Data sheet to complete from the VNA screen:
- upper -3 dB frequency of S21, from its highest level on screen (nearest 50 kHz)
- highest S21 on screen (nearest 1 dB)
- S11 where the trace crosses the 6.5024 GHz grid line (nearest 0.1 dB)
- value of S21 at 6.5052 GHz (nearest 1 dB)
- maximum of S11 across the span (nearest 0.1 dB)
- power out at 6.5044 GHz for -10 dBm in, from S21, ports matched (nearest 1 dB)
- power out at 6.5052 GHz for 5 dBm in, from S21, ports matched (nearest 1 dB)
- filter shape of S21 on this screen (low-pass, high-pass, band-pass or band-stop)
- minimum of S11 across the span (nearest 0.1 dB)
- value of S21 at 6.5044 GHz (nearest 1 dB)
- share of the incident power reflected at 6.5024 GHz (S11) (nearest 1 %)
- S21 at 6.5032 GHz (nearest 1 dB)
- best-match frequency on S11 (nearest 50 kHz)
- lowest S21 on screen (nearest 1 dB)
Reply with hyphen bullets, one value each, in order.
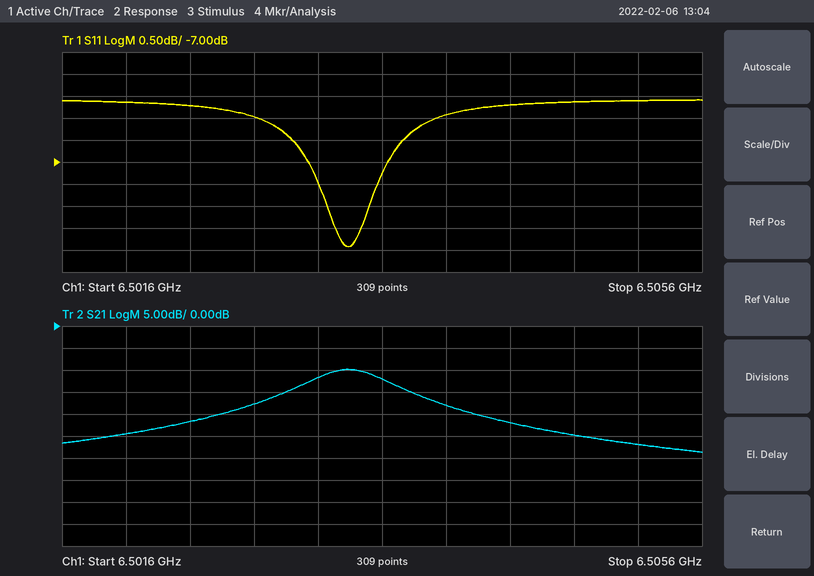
- 6.50365 GHz
- -10 dB
- -5.7 dB
- -27 dB
- -5.6 dB
- -32 dBm
- -22 dBm
- band-pass
- -8.9 dB
- -22 dB
- 27 %
- -12 dB
- 6.50340 GHz
- -29 dB
